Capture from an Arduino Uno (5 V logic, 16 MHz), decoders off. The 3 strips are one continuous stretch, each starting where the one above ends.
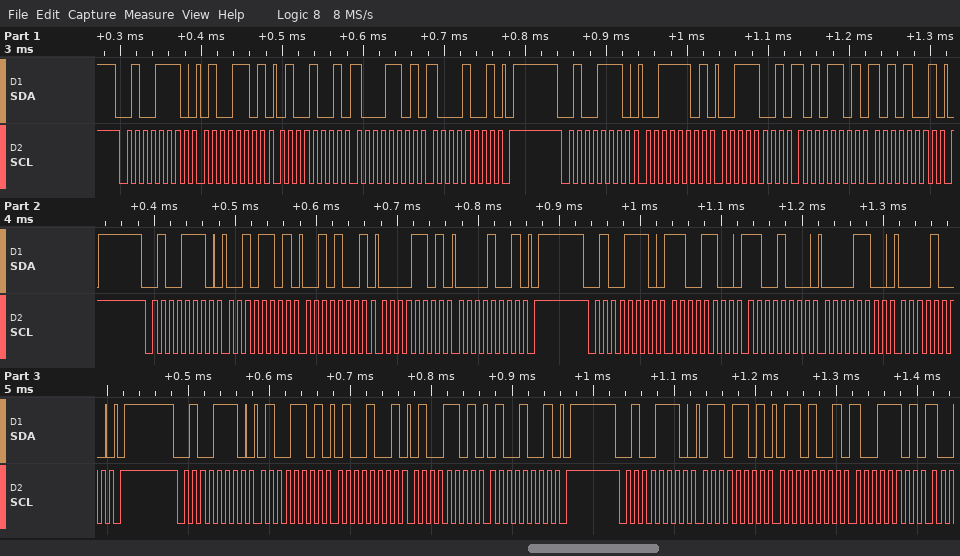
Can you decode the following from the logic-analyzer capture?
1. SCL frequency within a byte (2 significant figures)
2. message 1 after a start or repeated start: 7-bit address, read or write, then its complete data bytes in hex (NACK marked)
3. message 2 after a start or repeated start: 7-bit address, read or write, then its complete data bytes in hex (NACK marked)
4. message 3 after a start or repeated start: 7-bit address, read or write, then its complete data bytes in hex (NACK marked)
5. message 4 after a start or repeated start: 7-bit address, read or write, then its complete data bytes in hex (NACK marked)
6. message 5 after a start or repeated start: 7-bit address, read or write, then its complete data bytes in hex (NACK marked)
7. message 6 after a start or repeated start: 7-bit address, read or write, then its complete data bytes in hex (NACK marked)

100 kHz
0x27 write: 4D 49 8D 89
0x27 write: 3D 39 AD A9
0x27 write: 2D 29 0D 09
0x27 write: CC C8 0C 08
0x27 write: 4D 49 4D 49
0x27 write: 6D 69 9D
